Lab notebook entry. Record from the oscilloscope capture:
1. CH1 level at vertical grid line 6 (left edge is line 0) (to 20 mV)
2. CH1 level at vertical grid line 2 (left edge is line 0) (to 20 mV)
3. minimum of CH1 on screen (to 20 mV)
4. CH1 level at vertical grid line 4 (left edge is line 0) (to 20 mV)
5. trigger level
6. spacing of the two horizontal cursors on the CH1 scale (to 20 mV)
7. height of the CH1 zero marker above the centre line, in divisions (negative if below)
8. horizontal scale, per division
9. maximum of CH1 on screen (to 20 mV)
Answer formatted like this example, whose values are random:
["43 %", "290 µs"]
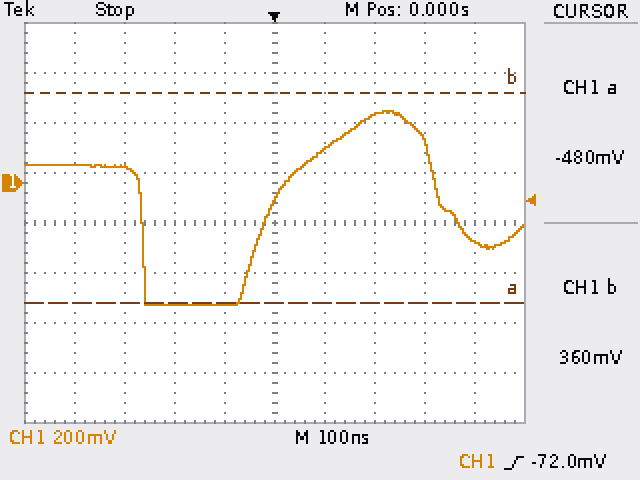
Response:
["140 mV", "60 mV", "-480 mV", "-480 mV", "-72.0 mV", "840 mV", "+0.8 div", "100 ns", "280 mV"]
